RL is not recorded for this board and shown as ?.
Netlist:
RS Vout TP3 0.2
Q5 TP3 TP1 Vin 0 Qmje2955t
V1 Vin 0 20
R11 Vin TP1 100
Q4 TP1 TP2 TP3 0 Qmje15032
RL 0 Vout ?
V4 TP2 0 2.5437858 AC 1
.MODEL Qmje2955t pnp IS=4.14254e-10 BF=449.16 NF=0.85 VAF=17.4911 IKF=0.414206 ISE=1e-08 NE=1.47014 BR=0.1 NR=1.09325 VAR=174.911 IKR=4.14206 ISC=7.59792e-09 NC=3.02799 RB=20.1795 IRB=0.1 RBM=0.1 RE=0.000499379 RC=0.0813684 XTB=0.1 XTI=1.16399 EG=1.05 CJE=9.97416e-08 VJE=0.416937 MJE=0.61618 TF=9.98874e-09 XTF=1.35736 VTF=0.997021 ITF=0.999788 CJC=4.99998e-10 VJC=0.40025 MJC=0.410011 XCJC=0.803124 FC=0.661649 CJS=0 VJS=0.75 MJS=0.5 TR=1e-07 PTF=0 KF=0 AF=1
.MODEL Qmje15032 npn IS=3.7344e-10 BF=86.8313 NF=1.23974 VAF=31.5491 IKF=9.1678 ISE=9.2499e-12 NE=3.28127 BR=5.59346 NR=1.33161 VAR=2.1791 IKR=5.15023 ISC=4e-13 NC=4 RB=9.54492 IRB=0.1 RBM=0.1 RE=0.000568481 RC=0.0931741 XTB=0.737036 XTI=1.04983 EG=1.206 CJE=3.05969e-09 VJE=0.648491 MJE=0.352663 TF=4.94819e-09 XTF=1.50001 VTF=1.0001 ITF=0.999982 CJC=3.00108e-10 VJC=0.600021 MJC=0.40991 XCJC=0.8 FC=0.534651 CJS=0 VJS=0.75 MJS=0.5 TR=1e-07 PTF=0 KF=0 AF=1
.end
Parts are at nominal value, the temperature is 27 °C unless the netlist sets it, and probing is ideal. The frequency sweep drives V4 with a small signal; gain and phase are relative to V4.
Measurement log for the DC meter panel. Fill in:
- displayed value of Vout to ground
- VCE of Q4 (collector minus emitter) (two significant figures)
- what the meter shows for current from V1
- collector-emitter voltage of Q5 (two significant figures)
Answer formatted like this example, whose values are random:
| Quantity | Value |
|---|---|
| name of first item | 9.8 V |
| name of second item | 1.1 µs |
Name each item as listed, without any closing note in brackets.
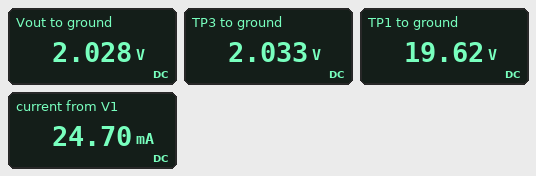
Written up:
| Quantity | Value |
|---|---|
| displayed value of Vout to ground | 2.028 V |
| VCE of Q4 (collector minus emitter) | 18 V |
| what the meter shows for current from V1 | 24.70 mA |
| collector-emitter voltage of Q5 | -18 V |
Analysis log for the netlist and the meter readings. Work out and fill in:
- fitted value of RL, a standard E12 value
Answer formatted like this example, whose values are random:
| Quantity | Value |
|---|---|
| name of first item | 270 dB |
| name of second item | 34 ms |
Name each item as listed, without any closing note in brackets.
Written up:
| Quantity | Value |
|---|---|
| fitted value of RL, a standard E12 value | 82 Ω |
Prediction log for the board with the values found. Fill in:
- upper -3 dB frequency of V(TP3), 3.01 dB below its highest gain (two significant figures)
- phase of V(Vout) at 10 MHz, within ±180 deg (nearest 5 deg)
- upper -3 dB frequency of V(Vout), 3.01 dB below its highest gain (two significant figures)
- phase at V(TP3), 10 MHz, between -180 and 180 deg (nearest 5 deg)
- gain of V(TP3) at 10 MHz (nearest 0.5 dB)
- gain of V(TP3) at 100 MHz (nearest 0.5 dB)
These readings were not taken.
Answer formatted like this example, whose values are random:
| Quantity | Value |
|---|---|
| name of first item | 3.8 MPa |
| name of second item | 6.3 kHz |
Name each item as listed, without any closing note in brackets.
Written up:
| Quantity | Value |
|---|---|
| upper -3 dB frequency of V(TP3), 3.01 dB below its highest gain | 66 MHz |
| phase of V(Vout) at 10 MHz, within ±180 deg | -5 deg |
| upper -3 dB frequency of V(Vout), 3.01 dB below its highest gain | 66 MHz |
| phase at V(TP3), 10 MHz, between -180 and 180 deg | -5 deg |
| gain of V(TP3) at 10 MHz | -1.0 dB |
| gain of V(TP3) at 100 MHz | -4.0 dB |
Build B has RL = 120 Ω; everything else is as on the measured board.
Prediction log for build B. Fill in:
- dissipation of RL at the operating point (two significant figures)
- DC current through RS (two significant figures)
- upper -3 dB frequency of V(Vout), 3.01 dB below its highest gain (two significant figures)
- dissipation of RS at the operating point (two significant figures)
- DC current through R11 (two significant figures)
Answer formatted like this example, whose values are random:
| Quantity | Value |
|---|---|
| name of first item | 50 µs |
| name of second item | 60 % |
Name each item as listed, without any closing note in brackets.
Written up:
| Quantity | Value |
|---|---|
| dissipation of RL at the operating point | 34 mW |
| DC current through RS | 17 mA |
| upper -3 dB frequency of V(Vout), 3.01 dB below its highest gain | 72 MHz |
| dissipation of RS at the operating point | 57 µW |
| DC current through R11 | 3.7 mA |
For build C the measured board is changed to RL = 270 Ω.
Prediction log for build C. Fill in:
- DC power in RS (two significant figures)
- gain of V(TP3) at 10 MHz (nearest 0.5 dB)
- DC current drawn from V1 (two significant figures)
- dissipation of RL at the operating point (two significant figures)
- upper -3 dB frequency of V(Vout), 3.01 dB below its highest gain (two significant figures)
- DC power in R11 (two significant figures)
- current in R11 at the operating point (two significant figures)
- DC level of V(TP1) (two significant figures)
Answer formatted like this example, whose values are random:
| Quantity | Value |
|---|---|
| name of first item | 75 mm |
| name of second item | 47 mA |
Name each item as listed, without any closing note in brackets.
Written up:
| Quantity | Value |
|---|---|
| DC power in RS | 11 µW |
| gain of V(TP3) at 10 MHz | -0.5 dB |
| DC current drawn from V1 | 7.5 mA |
| dissipation of RL at the operating point | 15 mW |
| upper -3 dB frequency of V(Vout), 3.01 dB below its highest gain | 79 MHz |
| DC power in R11 | 1.2 mW |
| current in R11 at the operating point | 3.4 mA |
| DC level of V(TP1) | 20 V |
